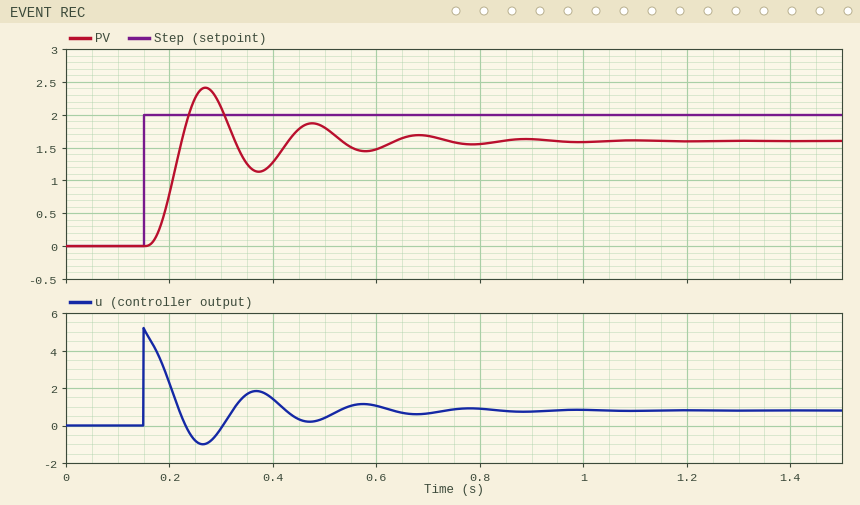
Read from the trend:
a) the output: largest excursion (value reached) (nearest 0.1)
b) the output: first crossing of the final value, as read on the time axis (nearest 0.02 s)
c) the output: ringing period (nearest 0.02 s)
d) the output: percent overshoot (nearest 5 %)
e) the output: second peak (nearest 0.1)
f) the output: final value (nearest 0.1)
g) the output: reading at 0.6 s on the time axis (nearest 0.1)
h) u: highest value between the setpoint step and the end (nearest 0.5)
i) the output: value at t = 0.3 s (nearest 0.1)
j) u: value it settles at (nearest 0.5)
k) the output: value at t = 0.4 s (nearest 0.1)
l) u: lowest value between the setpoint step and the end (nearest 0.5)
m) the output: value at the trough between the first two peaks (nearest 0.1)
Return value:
2.4
0.22 s
0.20 s
50 %
1.9
1.6
1.5
5.0
2.1
1.0
1.3
-1.0
1.1
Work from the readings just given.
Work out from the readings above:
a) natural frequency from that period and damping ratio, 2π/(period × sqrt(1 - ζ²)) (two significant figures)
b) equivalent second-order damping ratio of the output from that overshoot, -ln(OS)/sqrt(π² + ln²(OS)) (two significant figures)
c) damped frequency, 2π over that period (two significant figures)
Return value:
32 rad/s
0.22
31 rad/s
